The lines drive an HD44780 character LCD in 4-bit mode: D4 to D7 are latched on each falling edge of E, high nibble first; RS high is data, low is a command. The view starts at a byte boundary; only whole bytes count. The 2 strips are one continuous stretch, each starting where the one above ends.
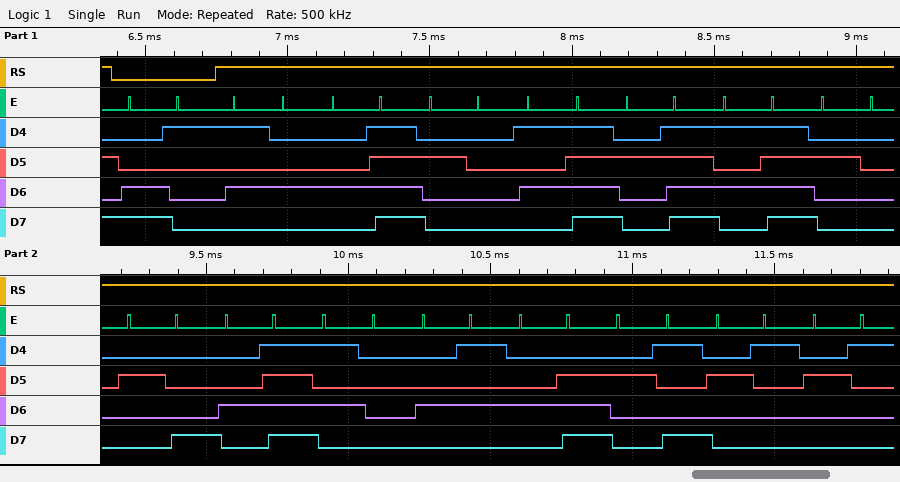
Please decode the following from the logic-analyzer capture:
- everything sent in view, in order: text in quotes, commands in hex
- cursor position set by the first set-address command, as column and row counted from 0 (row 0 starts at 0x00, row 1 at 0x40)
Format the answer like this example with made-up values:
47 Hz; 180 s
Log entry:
0xC1 "TO _/_ (OPEN)!!"; column 1, row 1
